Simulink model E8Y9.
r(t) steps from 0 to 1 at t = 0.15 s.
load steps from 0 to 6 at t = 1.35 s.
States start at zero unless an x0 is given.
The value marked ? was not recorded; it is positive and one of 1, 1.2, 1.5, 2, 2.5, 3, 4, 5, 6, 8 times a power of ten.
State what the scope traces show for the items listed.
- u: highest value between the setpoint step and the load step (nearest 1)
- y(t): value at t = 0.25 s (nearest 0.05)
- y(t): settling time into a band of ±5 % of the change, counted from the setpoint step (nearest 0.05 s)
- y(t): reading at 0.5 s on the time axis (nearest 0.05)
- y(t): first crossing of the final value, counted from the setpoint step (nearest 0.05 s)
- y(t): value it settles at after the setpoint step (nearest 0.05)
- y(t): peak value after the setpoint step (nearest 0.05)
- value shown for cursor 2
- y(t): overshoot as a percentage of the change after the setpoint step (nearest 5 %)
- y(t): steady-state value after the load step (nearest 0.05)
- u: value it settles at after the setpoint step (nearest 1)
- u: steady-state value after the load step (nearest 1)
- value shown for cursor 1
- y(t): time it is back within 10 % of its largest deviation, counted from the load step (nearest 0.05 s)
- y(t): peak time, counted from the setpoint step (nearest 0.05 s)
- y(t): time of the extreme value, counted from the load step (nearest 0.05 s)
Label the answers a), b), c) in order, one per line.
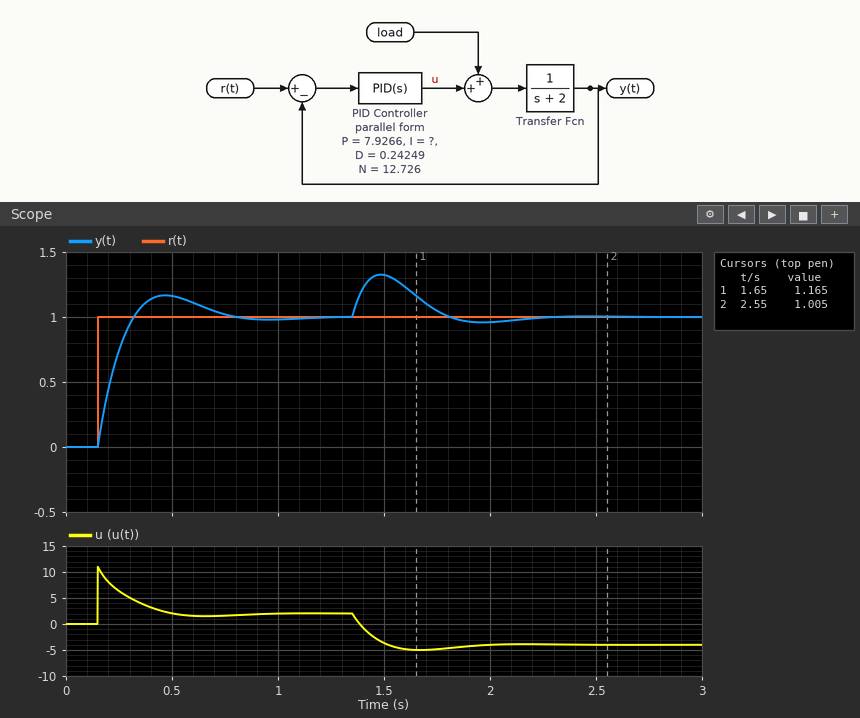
a) 11
b) 0.75
c) 0.55 s
d) 1.15
e) 0.15 s
f) 1.00
g) 1.15
h) 1.005
i) 15 %
j) 1.00
k) 2
l) -4
m) 1.165
n) 0.70 s
o) 0.30 s
p) 0.15 s
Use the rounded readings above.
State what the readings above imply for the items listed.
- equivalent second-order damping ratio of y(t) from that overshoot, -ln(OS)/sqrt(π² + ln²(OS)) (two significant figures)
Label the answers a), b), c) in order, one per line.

a) 0.52
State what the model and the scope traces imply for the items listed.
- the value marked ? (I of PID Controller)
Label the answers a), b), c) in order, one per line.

a) 80
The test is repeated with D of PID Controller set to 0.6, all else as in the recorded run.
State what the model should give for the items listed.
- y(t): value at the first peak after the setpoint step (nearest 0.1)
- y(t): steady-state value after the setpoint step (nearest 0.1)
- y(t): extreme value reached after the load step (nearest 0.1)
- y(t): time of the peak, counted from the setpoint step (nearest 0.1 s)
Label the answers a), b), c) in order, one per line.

a) 1.1
b) 1.0
c) 1.3
d) 0.4 s
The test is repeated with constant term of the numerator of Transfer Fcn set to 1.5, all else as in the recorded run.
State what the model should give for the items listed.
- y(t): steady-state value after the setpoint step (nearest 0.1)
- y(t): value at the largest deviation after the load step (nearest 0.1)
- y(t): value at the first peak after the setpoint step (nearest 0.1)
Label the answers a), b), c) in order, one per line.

a) 1.0
b) 1.4
c) 1.1
